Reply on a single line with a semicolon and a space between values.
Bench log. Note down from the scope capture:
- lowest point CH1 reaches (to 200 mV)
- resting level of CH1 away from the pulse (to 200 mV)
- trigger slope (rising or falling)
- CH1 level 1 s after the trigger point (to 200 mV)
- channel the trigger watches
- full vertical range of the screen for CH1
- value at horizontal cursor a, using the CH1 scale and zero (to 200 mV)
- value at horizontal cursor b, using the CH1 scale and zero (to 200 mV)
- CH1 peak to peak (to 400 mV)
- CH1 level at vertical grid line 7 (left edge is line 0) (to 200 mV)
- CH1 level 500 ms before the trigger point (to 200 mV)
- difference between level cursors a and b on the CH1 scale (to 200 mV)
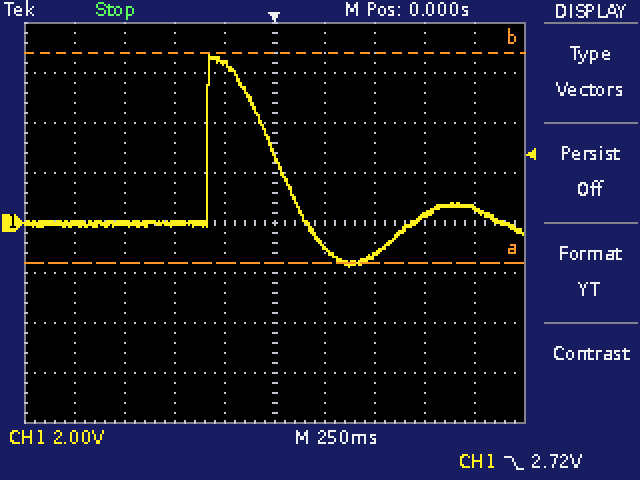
-1.8 V; 0.0 V; falling; 600 mV; CH1; 16 V; -1.6 V; 6.8 V; 8.4 V; -1.2 V; 0.0 V; 8.4 V
